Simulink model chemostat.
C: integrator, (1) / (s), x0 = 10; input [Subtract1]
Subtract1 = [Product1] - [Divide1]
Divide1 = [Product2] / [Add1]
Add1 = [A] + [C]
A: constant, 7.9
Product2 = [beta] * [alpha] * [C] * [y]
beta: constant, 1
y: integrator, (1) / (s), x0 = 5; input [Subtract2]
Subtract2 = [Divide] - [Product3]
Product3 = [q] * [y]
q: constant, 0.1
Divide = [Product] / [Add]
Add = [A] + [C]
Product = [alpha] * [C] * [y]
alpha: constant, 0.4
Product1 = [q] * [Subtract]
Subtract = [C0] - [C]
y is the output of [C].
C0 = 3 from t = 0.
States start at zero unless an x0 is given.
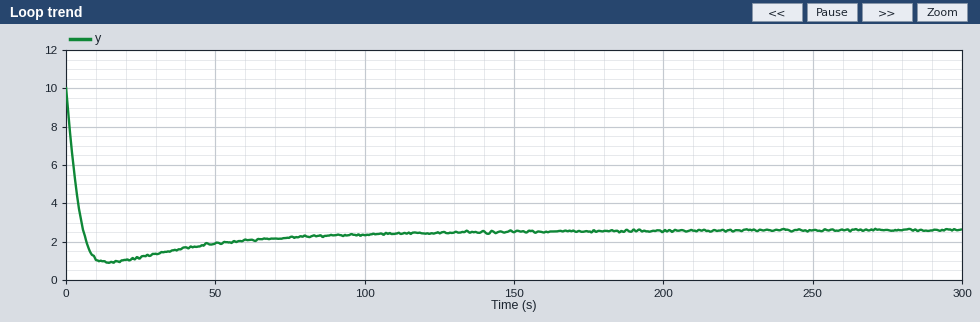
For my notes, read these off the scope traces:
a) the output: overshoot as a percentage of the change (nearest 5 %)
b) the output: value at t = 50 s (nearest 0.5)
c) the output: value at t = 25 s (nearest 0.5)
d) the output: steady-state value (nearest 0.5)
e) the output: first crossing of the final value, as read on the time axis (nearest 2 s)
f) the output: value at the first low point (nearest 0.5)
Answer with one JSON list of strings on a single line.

["25 %", "2.0", "1.0", "2.5", "6 s", "1.0"]
